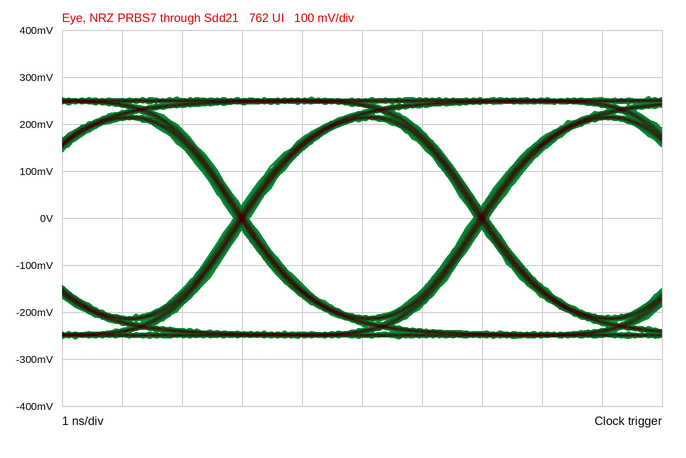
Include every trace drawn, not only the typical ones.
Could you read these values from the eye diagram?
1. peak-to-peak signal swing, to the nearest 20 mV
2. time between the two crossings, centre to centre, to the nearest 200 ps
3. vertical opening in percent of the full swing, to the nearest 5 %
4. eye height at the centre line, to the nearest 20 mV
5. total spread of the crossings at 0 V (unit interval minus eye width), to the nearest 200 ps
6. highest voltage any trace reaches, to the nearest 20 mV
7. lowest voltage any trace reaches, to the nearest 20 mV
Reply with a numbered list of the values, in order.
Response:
1. 520 mV
2. 4.0 ns
3. 80 %
4. 420 mV
5. 200 ps
6. 260 mV
7. -260 mV
